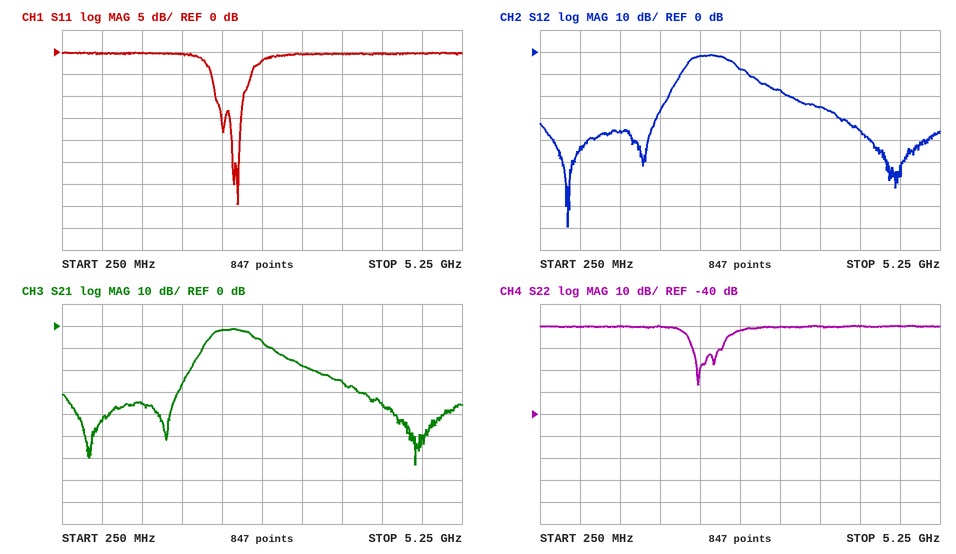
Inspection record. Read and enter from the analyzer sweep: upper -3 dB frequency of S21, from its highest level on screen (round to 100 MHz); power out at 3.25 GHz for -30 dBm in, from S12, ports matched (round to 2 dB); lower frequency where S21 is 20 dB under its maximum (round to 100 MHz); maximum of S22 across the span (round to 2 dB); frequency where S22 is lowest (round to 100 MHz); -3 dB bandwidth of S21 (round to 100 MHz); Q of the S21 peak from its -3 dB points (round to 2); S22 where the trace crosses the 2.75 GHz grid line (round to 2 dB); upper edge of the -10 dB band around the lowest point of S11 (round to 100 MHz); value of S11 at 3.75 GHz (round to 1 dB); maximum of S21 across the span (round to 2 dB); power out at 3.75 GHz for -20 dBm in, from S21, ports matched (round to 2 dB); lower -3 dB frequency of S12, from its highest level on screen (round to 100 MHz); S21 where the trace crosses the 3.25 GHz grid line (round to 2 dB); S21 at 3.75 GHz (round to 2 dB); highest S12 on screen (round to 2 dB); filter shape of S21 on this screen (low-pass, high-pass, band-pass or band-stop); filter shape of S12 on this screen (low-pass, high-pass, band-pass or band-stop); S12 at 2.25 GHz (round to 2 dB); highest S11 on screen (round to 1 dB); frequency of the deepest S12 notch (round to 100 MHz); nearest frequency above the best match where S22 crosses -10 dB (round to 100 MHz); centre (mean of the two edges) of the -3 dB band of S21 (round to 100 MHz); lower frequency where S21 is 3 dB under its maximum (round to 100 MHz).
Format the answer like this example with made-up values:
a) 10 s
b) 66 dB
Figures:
a) 2.6 GHz
b) -48 dBm
c) 1.8 GHz
d) 0 dB
e) 2.2 GHz
f) 500 MHz
g) 4
h) -2 dB
i) 2.5 GHz
j) 0 dB
k) -2 dB
l) -46 dBm
m) 2.1 GHz
n) -18 dB
o) -26 dB
p) -2 dB
q) band-pass
r) band-pass
s) -2 dB
t) 0 dB
u) 600 MHz
v) 2.5 GHz
w) 2.4 GHz
x) 2.1 GHz
